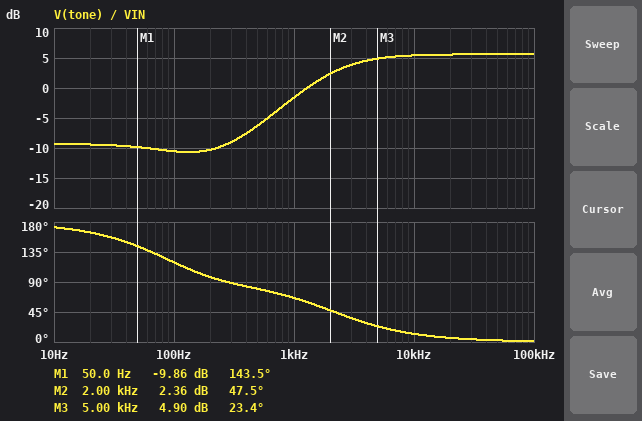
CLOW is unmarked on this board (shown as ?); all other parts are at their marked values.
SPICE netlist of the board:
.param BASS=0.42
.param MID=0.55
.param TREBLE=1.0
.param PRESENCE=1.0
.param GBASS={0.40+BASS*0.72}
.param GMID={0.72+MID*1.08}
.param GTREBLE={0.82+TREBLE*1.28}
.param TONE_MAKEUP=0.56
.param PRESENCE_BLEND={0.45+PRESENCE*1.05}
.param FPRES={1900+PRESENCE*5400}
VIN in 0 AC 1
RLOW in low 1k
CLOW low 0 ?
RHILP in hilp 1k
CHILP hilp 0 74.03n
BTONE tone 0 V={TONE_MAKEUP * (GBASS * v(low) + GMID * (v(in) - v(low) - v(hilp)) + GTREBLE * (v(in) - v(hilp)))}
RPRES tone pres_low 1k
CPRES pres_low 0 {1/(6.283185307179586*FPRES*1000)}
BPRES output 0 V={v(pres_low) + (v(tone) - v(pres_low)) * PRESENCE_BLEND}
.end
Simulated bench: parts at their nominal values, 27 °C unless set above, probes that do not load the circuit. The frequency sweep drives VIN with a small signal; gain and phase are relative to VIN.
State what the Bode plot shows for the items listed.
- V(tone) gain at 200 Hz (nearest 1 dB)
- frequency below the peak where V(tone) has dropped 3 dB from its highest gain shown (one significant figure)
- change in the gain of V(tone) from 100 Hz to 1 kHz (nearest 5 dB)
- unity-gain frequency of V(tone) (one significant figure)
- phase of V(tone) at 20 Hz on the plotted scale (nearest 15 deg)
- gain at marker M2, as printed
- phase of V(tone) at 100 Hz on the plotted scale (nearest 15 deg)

-10 dB
2 kHz
10 dB
1 kHz
165 deg
2.36 dB
120 deg
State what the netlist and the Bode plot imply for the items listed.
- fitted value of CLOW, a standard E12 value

1.8 µF
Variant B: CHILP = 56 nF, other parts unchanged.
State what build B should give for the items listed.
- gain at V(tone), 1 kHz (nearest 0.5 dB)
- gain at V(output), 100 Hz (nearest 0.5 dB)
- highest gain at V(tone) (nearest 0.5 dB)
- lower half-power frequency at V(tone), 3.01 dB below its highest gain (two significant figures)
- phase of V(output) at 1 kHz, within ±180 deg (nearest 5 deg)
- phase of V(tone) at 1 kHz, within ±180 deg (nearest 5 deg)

-3.5 dB
-11.0 dB
5.5 dB
2.8 kHz
75 deg
70 deg
